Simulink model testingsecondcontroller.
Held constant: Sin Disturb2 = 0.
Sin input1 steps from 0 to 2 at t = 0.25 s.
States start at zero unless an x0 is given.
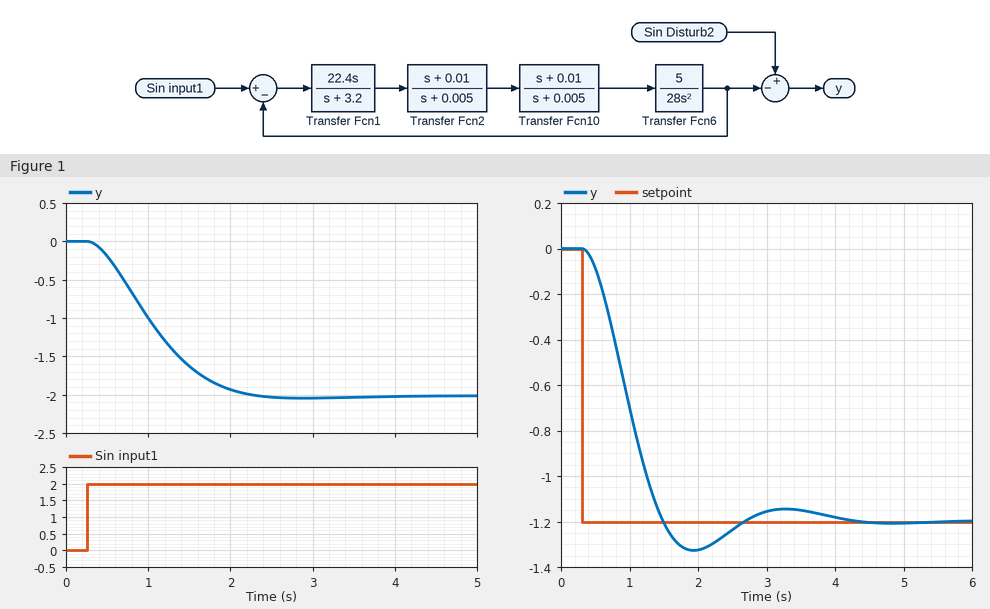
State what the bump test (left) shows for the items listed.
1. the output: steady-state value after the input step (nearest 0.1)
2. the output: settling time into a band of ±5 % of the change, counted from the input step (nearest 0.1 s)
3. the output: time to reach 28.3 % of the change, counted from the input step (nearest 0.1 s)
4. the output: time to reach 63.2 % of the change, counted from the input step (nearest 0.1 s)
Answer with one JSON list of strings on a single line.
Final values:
["-2.0", "1.7 s", "0.5 s", "0.9 s"]
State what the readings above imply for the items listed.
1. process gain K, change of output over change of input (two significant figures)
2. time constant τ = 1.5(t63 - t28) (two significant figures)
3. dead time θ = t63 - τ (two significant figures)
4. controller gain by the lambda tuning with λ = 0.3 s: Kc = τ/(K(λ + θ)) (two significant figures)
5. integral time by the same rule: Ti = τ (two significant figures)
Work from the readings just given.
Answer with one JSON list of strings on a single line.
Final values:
["-1.0", "0.60 s", "0.30 s", "-1.0", "0.60 s"]
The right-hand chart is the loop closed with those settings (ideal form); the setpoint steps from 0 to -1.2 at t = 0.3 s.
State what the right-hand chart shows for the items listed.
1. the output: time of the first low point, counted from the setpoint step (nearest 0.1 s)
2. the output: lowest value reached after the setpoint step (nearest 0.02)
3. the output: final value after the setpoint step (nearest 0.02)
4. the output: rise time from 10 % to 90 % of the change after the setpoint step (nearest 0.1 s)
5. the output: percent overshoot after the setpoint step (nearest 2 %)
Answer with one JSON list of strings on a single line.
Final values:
["1.6 s", "-1.32", "-1.20", "0.8 s", "10 %"]
